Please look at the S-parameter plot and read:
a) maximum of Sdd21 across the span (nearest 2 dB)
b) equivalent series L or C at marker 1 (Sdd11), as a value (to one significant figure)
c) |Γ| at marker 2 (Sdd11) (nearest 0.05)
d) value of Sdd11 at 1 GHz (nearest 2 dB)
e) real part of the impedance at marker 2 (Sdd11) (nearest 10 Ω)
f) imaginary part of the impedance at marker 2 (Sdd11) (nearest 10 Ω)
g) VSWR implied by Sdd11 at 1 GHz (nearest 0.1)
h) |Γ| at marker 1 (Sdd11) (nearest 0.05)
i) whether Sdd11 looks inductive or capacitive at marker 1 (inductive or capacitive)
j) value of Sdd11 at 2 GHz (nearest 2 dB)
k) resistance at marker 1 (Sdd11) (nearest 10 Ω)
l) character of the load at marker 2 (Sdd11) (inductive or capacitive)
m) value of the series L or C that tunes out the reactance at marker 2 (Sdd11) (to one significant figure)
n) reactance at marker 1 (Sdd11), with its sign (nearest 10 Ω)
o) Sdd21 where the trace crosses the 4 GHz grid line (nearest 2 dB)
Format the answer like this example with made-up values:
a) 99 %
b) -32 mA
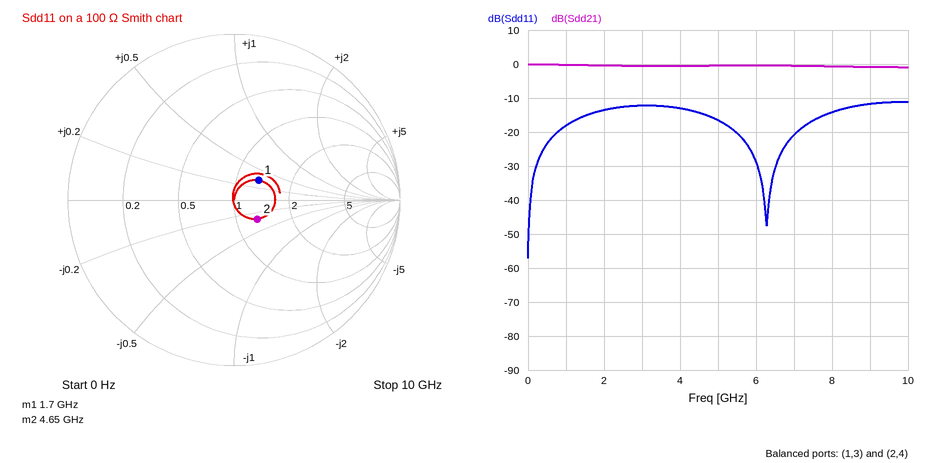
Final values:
a) 0 dB
b) 3 nH
c) 0.20
d) -18 dB
e) 130 Ω
f) -30 Ω
g) 1.3
h) 0.20
i) inductive
j) -14 dB
k) 130 Ω
l) capacitive
m) 1 nH
n) +30 Ω
o) 0 dB
